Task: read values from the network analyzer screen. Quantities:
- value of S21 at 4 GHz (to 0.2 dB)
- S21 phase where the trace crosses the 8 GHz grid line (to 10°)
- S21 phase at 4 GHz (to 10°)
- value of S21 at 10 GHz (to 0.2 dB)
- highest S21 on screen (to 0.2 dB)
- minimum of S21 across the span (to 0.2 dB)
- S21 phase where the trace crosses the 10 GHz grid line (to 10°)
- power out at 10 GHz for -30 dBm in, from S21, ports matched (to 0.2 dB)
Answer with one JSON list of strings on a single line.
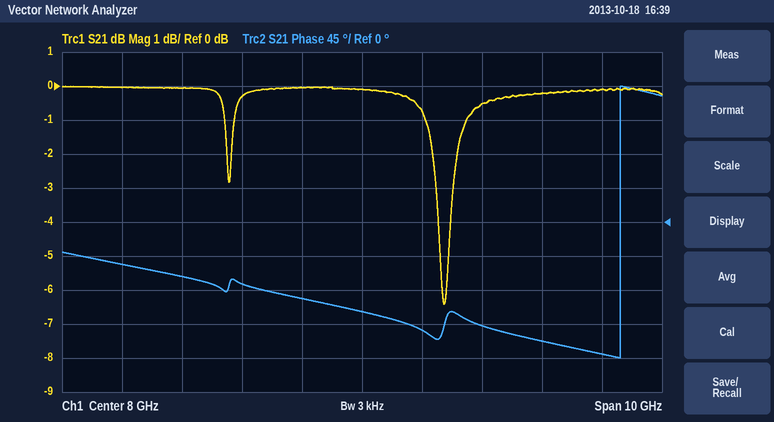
["0.0 dB", "-120°", "-60°", "-0.6 dB", "0.0 dB", "-6.4 dB", "-140°", "-30.6 dBm"]
